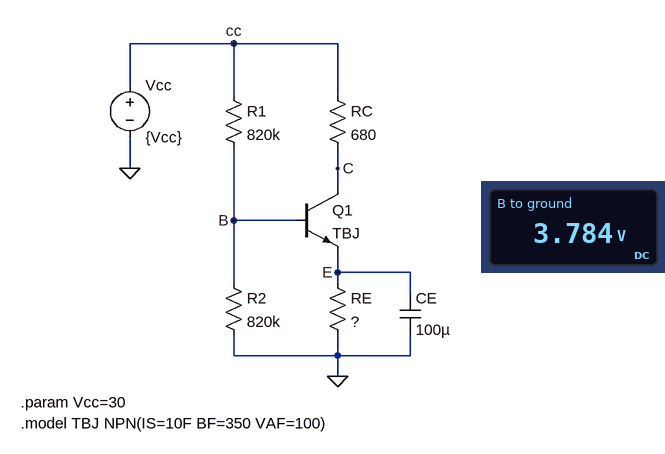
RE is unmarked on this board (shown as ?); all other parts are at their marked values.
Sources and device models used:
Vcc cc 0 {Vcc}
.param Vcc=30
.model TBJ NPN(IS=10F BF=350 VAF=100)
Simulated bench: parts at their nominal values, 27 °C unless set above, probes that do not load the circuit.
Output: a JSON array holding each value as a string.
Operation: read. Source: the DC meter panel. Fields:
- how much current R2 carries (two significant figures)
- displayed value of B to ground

["4.6 µA", "3.784 V"]
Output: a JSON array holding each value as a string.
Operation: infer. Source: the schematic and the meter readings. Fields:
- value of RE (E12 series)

["270 Ω"]
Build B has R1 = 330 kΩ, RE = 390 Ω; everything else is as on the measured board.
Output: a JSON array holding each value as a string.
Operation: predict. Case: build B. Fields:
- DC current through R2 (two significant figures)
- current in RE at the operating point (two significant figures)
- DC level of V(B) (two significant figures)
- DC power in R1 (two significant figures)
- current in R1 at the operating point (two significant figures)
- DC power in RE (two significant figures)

["11 µA", "20 mA", "8.7 V", "1.4 mW", "65 µA", "160 mW"]
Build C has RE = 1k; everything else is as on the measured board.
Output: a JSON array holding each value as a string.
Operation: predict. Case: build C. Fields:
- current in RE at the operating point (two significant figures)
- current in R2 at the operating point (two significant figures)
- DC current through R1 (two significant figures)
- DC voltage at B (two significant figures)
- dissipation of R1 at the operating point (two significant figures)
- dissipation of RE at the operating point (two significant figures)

["7.2 mA", "9.6 µA", "27 µA", "7.9 V", "600 µW", "51 mW"]
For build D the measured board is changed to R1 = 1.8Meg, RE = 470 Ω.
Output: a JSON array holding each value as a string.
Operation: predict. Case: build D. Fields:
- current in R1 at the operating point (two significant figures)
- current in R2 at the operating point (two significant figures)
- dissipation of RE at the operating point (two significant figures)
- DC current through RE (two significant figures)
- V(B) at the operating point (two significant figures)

["15 µA", "3.7 µA", "11 mW", "4.9 mA", "3.0 V"]
